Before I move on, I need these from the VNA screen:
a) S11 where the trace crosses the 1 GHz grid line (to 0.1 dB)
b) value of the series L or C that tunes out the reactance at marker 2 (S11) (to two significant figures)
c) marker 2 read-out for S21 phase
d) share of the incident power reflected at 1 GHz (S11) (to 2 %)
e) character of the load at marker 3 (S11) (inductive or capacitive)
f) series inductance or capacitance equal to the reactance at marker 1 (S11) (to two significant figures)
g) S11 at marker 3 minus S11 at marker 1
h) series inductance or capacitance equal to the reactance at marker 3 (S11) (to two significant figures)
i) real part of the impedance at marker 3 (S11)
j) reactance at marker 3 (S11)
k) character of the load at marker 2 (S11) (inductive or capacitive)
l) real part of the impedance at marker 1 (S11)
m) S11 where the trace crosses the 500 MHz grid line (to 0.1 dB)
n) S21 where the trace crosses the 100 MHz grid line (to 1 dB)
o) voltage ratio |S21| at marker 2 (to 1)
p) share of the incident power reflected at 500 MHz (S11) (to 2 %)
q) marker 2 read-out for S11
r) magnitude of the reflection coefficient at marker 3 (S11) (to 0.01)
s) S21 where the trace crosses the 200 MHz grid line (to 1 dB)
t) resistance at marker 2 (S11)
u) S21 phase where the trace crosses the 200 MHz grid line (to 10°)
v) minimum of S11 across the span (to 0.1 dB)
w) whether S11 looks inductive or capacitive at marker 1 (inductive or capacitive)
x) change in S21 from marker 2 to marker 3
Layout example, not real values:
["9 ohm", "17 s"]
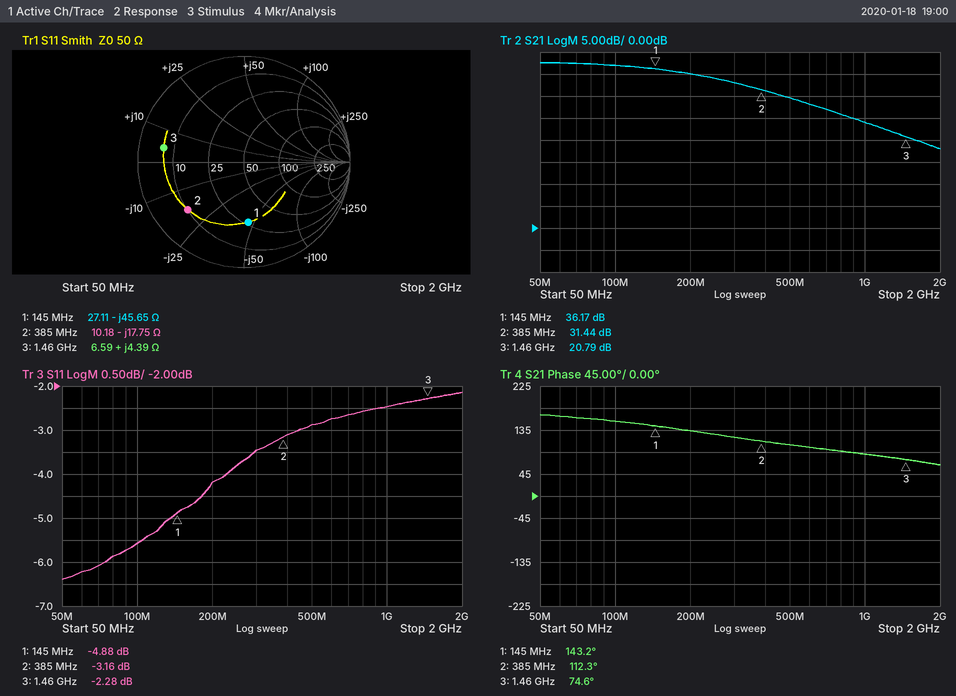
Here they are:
["-2.5 dB", "7.3 nH", "112.3°", "56 %", "inductive", "24 pF", "2.60 dB", "480 pH", "6.59 Ω", "+4.39 Ω", "capacitive", "27.11 Ω", "-2.9 dB", "37 dB", "37", "52 %", "-3.16 dB", "0.77", "35 dB", "10.18 Ω", "130°", "-6.4 dB", "capacitive", "-10.65 dB"]
